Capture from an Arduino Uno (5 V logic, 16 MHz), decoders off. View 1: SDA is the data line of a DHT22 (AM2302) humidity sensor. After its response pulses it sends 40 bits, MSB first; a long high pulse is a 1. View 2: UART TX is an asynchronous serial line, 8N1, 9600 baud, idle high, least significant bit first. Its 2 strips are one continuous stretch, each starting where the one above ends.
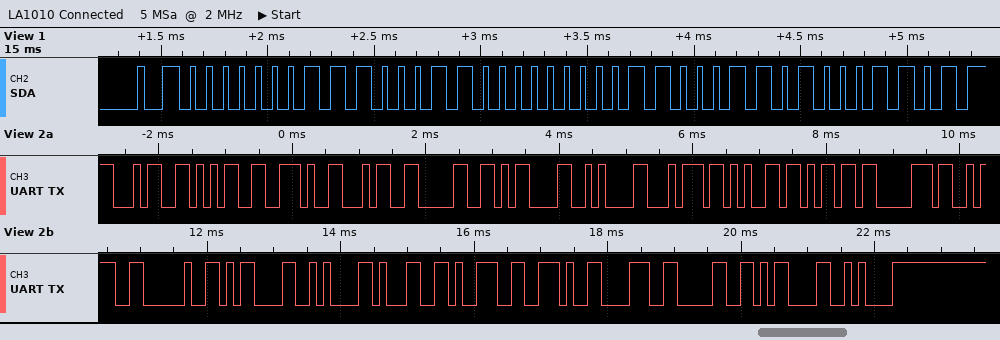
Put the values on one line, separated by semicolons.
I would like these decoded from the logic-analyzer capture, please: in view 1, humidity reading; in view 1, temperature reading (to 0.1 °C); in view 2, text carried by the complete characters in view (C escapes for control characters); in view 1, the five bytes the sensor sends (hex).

45.4 %; 19.8 °C; "45.40\r\ntemp: \r\n19.80\r\n"; 01 C6 00 C6 8D
